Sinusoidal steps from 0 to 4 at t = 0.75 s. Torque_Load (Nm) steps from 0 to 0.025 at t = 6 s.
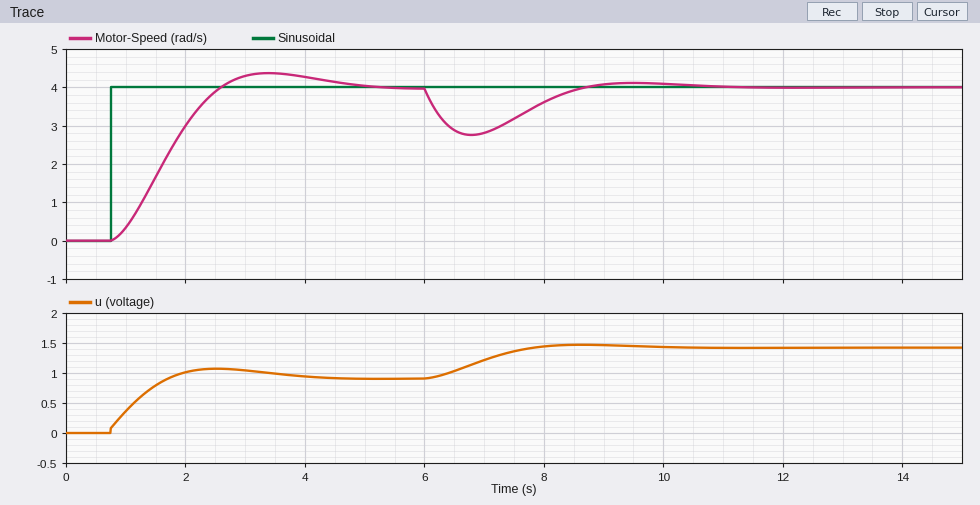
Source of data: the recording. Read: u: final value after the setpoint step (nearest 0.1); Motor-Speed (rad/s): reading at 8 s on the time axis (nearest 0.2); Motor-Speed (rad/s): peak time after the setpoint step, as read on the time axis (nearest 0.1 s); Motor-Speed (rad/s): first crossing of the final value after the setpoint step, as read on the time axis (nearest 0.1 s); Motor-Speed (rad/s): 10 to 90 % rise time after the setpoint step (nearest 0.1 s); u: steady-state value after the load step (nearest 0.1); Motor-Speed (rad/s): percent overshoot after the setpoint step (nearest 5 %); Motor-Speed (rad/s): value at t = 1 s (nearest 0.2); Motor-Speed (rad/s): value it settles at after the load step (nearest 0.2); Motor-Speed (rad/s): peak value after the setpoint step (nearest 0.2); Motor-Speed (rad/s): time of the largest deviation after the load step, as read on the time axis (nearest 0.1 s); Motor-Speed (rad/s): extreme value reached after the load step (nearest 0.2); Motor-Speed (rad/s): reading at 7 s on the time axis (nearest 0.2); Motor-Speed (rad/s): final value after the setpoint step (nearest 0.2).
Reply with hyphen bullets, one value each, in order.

- 0.9
- 3.6
- 3.4 s
- 2.6 s
- 1.3 s
- 1.4
- 10 %
- 0.4
- 4.0
- 4.4
- 6.8 s
- 2.8
- 2.8
- 4.0
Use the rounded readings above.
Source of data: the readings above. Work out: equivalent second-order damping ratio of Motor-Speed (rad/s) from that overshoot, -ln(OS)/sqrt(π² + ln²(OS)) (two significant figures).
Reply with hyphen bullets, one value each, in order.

- 0.59
